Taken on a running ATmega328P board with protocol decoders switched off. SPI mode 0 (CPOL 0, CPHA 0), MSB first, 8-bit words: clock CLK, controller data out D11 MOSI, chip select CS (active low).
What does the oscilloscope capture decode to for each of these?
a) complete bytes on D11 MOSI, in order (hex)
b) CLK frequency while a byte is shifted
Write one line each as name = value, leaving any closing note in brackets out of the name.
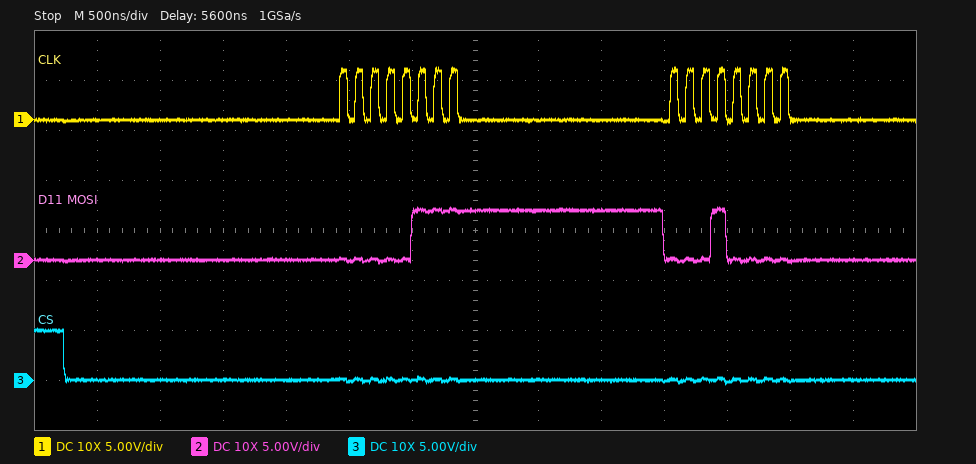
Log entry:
complete bytes on D11 MOSI, in order = 0x07 0x10
CLK frequency while a byte is shifted = 8 MHz
